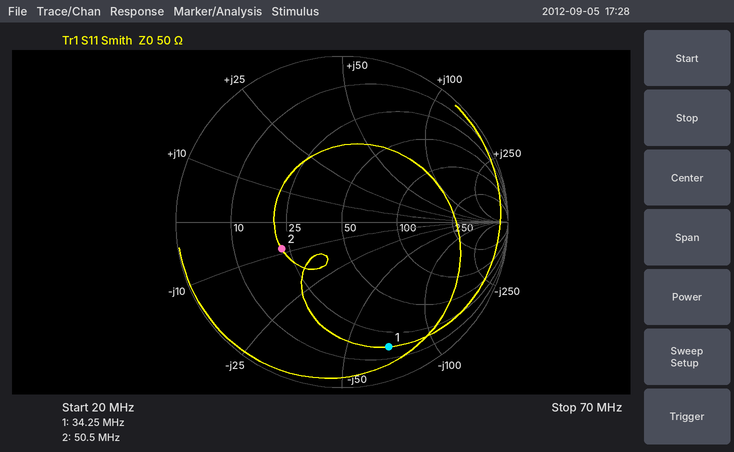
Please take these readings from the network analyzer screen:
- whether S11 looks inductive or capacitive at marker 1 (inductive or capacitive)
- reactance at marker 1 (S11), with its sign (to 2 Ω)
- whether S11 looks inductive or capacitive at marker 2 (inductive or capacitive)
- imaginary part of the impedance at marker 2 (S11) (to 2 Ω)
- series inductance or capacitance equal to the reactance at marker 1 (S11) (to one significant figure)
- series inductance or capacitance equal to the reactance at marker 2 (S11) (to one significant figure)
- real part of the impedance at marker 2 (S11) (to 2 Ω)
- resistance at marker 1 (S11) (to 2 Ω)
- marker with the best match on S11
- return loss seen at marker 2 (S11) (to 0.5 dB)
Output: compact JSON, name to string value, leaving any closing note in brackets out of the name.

{"whether S11 looks inductive or capacitive at marker 1": "capacitive", "reactance at marker 1 (S11), with its sign": "-70 Ω", "whether S11 looks inductive or capacitive at marker 2": "capacitive", "imaginary part of the impedance at marker 2 (S11)": "-8 Ω", "series inductance or capacitance equal to the reactance at marker 1 (S11)": "70 pF", "series inductance or capacitance equal to the reactance at marker 2 (S11)": "400 pF", "real part of the impedance at marker 2 (S11)": "22 Ω", "resistance at marker 1 (S11)": "16 Ω", "marker with the best match on S11": "marker 2", "return loss seen at marker 2 (S11)": "8.0 dB"}
